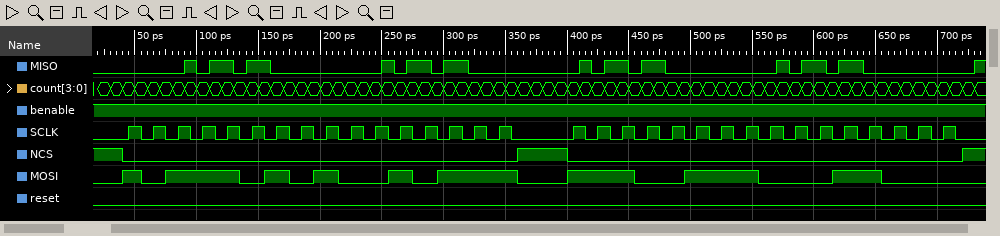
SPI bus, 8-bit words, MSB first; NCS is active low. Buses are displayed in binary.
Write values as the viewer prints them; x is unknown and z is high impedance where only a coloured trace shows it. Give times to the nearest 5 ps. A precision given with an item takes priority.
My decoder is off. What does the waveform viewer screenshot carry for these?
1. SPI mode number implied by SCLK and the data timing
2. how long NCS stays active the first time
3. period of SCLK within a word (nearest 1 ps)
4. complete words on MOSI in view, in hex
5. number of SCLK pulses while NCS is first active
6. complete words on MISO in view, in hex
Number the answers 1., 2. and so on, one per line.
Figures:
1. 0
2. 320 ps
3. 20 ps
4. BA, 97, E7, 18
5. 16
6. 0C, 0C, 30, 30
